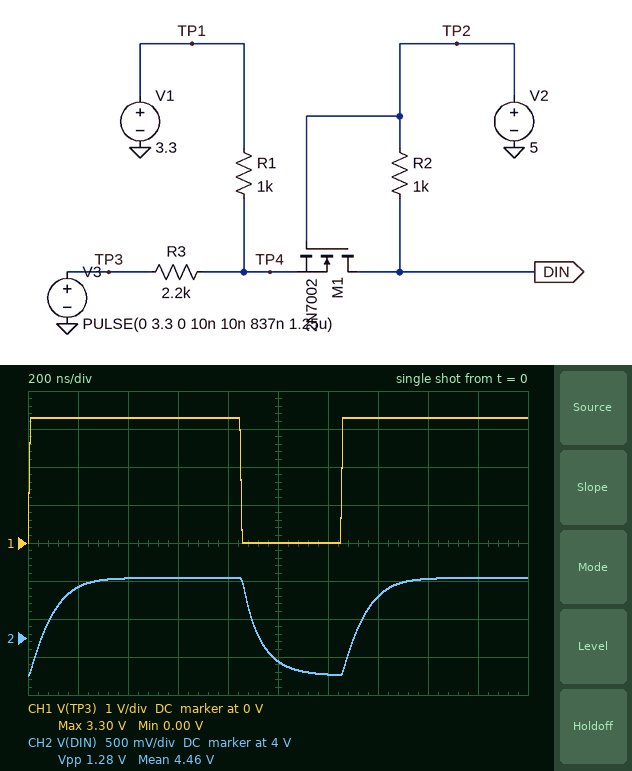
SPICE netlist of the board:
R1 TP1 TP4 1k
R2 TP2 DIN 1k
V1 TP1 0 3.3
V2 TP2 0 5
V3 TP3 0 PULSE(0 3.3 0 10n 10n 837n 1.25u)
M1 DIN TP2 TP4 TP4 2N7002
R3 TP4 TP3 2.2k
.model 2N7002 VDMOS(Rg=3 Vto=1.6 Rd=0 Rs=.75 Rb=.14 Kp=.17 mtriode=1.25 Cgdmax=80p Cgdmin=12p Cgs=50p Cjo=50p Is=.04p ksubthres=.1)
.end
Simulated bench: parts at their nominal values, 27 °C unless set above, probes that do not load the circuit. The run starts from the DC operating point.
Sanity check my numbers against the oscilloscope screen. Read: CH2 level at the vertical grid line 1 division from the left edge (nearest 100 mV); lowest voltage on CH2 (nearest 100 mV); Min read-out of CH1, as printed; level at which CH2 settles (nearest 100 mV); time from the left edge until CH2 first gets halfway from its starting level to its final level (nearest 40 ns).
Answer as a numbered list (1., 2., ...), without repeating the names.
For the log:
1. 4.7 V
2. 3.5 V
3. 0.00 V
4. 4.8 V
5. 80 ns
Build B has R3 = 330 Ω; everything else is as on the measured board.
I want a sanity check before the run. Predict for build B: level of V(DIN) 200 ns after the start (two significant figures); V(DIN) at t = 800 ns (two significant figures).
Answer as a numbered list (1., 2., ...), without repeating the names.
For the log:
1. 4.3 V
2. 4.6 V
